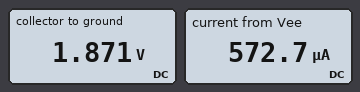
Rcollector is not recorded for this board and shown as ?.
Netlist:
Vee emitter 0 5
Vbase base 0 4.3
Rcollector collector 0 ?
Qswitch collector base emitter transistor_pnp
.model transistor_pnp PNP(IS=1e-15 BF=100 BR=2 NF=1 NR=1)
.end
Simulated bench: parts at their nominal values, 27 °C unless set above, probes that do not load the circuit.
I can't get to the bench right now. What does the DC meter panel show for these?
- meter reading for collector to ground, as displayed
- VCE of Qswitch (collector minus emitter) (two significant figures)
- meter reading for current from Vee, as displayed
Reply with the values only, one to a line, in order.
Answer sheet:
1.871 V
-3.1 V
572.7 µA
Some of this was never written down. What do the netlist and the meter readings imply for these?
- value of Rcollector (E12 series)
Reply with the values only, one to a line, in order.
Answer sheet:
3.3 kΩ
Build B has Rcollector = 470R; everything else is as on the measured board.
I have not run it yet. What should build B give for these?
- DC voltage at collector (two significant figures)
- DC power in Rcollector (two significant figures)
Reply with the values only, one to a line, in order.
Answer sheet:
270 mV
150 µW
